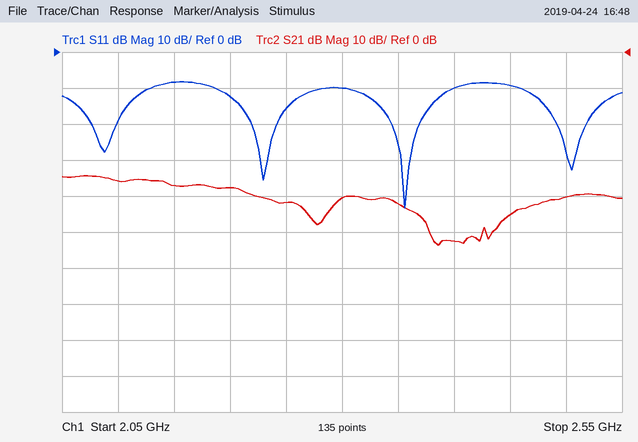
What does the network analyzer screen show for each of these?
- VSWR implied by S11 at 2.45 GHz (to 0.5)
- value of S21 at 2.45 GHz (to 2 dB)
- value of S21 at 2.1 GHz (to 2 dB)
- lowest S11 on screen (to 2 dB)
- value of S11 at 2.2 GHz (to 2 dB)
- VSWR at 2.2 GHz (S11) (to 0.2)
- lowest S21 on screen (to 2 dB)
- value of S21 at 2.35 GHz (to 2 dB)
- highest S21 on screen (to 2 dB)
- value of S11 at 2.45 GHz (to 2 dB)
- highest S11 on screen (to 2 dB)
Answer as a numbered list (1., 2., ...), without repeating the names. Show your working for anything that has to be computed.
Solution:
1. |Γ| = 10^(-10/20) = 0.3162; VSWR = (1 + 0.3162)/(1 − 0.3162) ≈ 1.92, so 2.0 to the nearest 0.5
2. -46 dB
3. -36 dB
4. -44 dB
5. -12 dB
6. |Γ| = 10^(-12/20) = 0.2512; VSWR = (1 + 0.2512)/(1 − 0.2512) ≈ 1.67, so 1.6 to the nearest 0.2
7. -54 dB
8. -42 dB
9. -34 dB
10. -10 dB
11. -8 dB
